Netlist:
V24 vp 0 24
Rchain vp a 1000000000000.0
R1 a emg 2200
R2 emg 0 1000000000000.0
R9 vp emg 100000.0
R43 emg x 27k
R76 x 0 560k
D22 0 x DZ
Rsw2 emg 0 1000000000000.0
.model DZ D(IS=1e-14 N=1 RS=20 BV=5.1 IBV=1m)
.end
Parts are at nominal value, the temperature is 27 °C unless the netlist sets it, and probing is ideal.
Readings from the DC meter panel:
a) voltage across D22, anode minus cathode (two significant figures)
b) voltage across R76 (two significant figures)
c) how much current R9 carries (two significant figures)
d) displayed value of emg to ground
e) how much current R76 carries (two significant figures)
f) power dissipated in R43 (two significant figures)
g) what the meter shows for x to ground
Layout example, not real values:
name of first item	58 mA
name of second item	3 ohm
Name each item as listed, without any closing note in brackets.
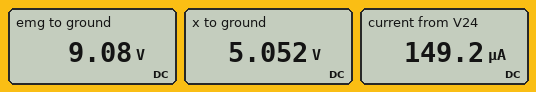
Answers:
voltage across D22, anode minus cathode	-5.1 V
voltage across R76	5.1 V
how much current R9 carries	150 µA
displayed value of emg to ground	9.08 V
how much current R76 carries	9.0 µA
power dissipated in R43	600 µW
what the meter shows for x to ground	5.052 V
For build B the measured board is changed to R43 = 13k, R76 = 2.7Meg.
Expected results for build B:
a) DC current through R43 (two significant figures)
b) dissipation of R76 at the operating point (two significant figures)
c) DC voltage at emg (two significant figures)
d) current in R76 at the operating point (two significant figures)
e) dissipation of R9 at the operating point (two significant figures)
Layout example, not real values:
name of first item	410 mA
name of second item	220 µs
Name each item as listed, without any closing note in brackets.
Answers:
DC current through R43	170 µA
dissipation of R76 at the operating point	9.5 µW
DC voltage at emg	7.2 V
current in R76 at the operating point	1.9 µA
dissipation of R9 at the operating point	2.8 mW
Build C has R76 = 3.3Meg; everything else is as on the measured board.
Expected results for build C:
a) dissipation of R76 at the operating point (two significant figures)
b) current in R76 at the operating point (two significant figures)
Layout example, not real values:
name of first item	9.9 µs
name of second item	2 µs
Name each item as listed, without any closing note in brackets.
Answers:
dissipation of R76 at the operating point	7.7 µW
current in R76 at the operating point	1.5 µA
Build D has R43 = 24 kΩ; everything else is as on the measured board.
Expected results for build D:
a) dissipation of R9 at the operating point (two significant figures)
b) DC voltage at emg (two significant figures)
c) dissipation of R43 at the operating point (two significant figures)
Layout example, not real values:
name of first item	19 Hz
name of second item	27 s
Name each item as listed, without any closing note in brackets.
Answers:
dissipation of R9 at the operating point	2.3 mW
DC voltage at emg	8.7 V
dissipation of R43 at the operating point	560 µW
